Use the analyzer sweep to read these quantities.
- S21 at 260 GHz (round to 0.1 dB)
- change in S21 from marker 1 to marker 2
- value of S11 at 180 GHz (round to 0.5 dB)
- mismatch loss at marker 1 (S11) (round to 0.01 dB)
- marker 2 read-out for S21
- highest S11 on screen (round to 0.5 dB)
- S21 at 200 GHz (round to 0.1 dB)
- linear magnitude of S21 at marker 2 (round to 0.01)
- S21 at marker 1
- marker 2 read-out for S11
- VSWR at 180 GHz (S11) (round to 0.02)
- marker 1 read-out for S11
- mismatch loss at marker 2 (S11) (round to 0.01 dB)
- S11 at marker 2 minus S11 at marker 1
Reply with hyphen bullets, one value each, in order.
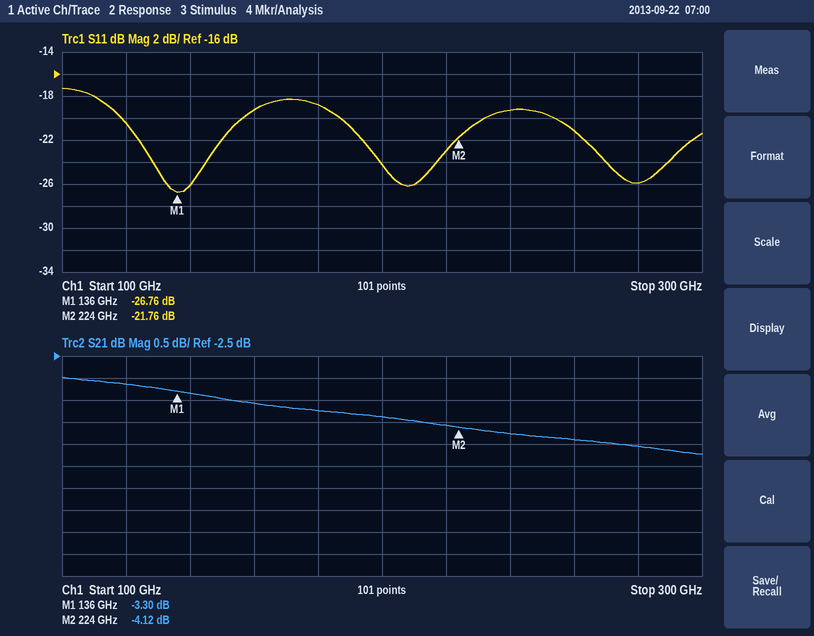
- -4.4 dB
- -0.82 dB
- -19.0 dB
- 0.01 dB
- -4.12 dB
- -17.5 dB
- -3.9 dB
- 0.62
- -3.30 dB
- -21.76 dB
- 1.26
- -26.76 dB
- 0.03 dB
- 5.00 dB
